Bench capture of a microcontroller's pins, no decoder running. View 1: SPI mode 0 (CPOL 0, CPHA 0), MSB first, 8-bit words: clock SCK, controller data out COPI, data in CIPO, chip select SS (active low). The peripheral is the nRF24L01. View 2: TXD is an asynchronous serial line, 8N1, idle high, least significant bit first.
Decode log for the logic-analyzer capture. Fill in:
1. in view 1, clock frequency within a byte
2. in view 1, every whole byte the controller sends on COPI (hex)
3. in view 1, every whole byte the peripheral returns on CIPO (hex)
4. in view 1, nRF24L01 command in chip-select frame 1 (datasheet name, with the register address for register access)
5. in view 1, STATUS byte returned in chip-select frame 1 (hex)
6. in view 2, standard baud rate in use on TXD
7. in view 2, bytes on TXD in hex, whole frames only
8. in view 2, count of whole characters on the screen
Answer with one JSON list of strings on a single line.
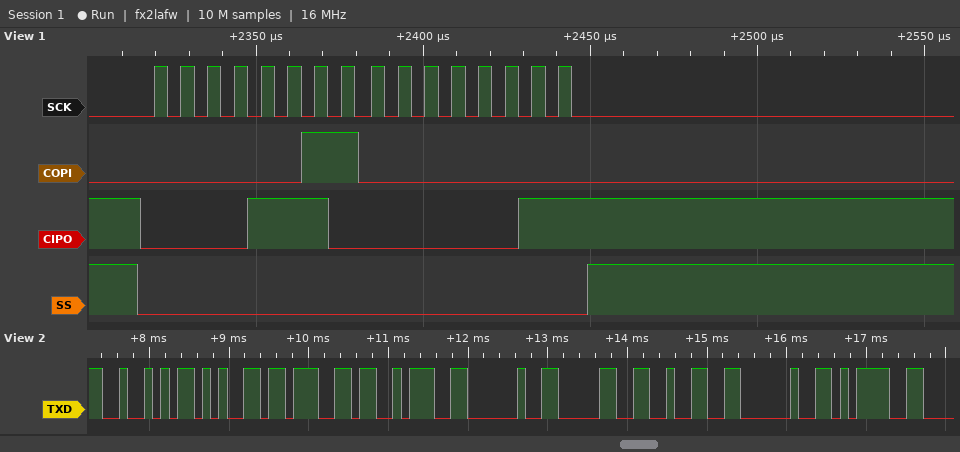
["125 kHz", "03 00", "0E 03", "R_REGISTER 0x03", "0x0E", "9600 baud", "0x52 0x65 0x67 0x3A 0x20 0x30 0x32 0x20 0x3D", "9"]
